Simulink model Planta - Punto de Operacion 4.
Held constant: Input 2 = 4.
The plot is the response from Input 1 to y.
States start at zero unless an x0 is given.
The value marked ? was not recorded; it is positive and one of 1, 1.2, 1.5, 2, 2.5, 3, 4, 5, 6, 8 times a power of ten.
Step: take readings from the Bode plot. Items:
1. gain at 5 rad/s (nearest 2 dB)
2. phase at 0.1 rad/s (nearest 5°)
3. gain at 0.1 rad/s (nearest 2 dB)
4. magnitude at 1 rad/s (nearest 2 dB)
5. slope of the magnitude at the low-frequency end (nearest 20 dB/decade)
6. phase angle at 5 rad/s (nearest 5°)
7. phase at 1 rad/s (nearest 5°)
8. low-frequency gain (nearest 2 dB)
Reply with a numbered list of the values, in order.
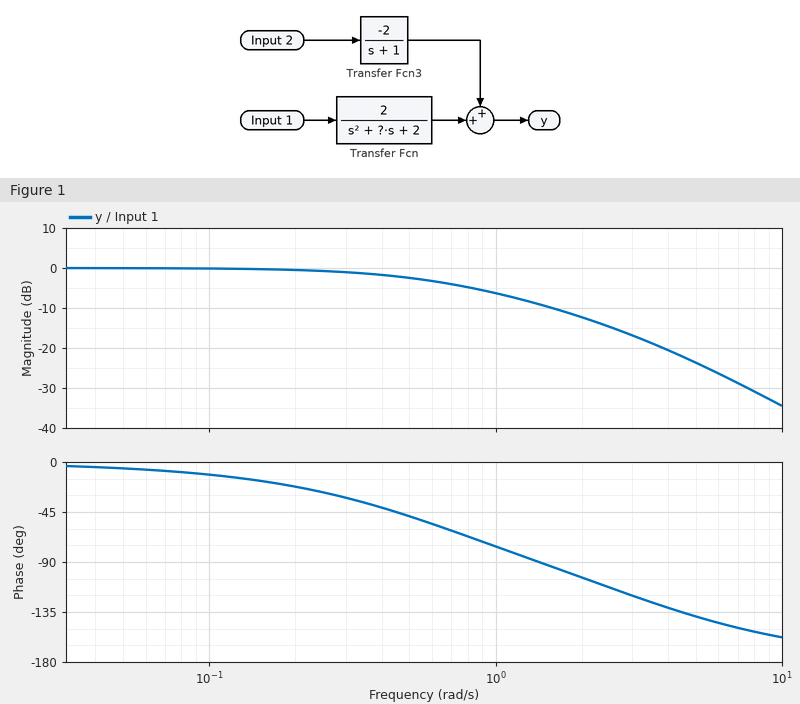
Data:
1. -24 dB
2. -10°
3. 0 dB
4. -6 dB
5. 0 dB/decade
6. -140°
7. -75°
8. 0 dB
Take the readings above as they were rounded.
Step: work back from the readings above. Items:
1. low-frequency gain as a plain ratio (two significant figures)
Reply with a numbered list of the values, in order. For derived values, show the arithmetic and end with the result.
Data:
1. 10^(0 / 20) = 1.0
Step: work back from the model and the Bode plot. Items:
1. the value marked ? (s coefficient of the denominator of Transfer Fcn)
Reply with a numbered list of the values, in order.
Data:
1. 4
